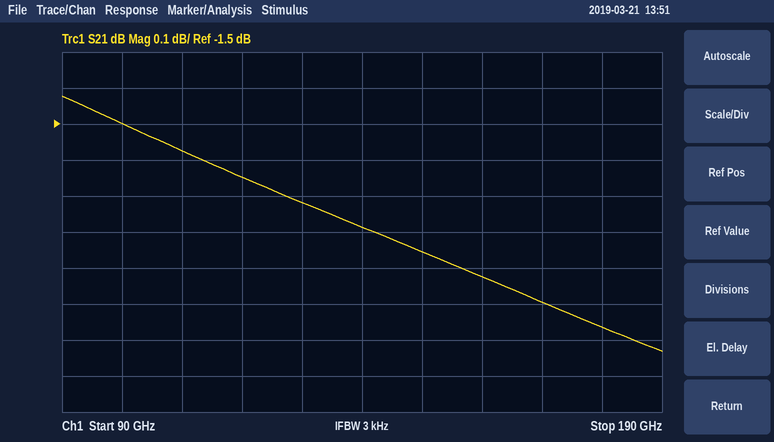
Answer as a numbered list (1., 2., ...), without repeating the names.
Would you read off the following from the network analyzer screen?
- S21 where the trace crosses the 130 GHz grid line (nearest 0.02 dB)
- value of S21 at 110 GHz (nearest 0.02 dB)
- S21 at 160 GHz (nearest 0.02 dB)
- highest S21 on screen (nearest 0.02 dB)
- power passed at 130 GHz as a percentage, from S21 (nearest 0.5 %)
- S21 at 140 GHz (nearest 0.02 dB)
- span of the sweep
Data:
1. -1.72 dB
2. -1.58 dB
3. -1.92 dB
4. -1.42 dB
5. 67.5 %
6. -1.78 dB
7. 100 GHz
